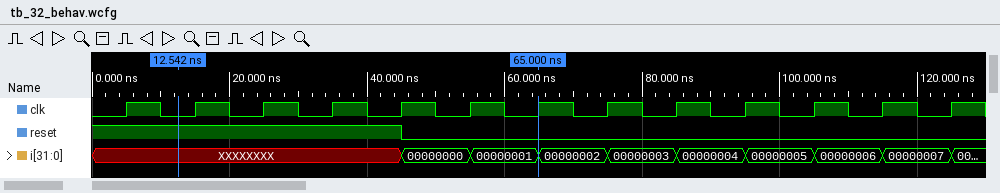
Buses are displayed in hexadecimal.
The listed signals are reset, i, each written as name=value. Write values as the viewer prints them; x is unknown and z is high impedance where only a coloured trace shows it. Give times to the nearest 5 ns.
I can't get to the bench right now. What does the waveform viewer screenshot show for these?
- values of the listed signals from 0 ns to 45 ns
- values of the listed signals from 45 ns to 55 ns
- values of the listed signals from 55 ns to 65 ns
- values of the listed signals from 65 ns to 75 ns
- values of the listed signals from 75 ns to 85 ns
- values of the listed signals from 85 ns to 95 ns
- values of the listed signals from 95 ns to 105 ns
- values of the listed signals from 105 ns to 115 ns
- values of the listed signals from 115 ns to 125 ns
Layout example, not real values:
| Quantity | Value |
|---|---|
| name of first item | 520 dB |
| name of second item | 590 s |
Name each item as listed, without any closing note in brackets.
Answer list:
| Quantity | Value |
|---|---|
| values of the listed signals from 0 ns to 45 ns | reset=1, i=XXXXXXXX |
| values of the listed signals from 45 ns to 55 ns | reset=0, i=00000000 |
| values of the listed signals from 55 ns to 65 ns | reset=0, i=00000001 |
| values of the listed signals from 65 ns to 75 ns | reset=0, i=00000002 |
| values of the listed signals from 75 ns to 85 ns | reset=0, i=00000003 |
| values of the listed signals from 85 ns to 95 ns | reset=0, i=00000004 |
| values of the listed signals from 95 ns to 105 ns | reset=0, i=00000005 |
| values of the listed signals from 105 ns to 115 ns | reset=0, i=00000006 |
| values of the listed signals from 115 ns to 125 ns | reset=0, i=00000007 |
